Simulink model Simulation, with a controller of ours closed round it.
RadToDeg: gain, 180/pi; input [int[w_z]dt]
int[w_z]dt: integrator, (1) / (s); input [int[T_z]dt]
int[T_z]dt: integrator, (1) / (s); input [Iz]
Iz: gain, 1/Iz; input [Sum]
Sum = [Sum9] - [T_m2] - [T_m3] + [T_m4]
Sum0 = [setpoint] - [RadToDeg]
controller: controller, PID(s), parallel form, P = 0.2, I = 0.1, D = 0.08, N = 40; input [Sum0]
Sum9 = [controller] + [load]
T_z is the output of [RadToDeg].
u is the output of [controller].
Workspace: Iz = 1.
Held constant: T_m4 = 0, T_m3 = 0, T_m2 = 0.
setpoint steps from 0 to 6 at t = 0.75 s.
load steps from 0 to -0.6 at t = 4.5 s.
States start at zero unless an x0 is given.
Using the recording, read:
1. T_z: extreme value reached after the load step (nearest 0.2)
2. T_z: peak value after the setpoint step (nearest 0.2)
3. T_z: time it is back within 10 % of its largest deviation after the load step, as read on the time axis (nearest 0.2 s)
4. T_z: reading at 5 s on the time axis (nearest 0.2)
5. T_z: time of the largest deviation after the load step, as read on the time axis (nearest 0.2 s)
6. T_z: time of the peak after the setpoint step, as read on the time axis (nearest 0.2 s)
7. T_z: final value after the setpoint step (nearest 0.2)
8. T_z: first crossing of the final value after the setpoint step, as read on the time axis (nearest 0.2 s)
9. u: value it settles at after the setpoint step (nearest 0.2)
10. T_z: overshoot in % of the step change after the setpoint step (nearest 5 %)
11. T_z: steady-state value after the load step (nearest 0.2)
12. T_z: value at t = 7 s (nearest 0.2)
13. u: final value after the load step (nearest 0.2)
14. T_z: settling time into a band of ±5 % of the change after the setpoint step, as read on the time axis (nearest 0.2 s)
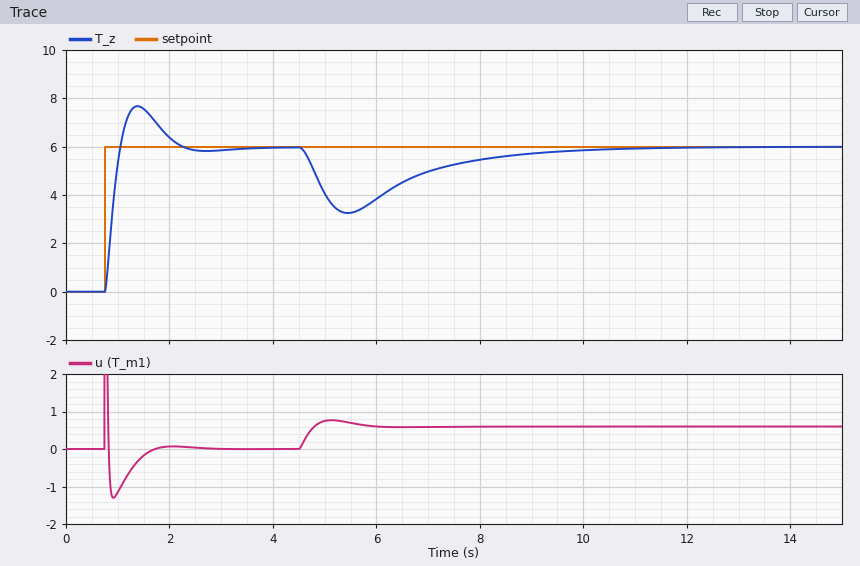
3.2
7.6
9.0 s
4.0
5.4 s
1.4 s
6.0
1.0 s
0.0
30 %
6.0
5.0
0.6
2.0 s
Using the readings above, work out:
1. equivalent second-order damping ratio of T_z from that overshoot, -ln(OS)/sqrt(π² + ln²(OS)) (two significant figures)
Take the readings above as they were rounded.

0.36
